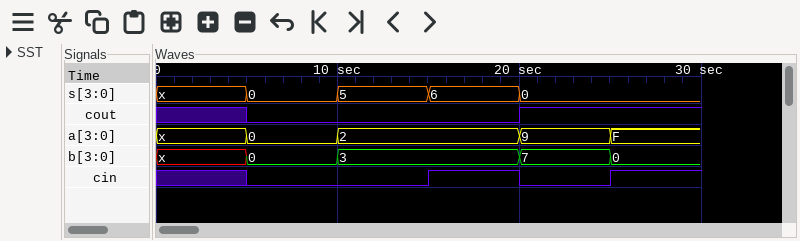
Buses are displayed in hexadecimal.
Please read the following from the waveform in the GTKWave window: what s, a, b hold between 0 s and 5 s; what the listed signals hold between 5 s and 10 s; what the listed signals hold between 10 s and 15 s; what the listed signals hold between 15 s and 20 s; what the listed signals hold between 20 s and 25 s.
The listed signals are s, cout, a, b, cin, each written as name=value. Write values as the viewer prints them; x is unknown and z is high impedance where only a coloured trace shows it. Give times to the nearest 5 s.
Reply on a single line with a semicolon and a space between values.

s=x, a=x, b=x; s=0, cout=0, a=0, b=0, cin=0; s=5, cout=0, a=2, b=3, cin=0; s=6, cout=0, a=2, b=3, cin=1; s=0, cout=1, a=9, b=7, cin=0
